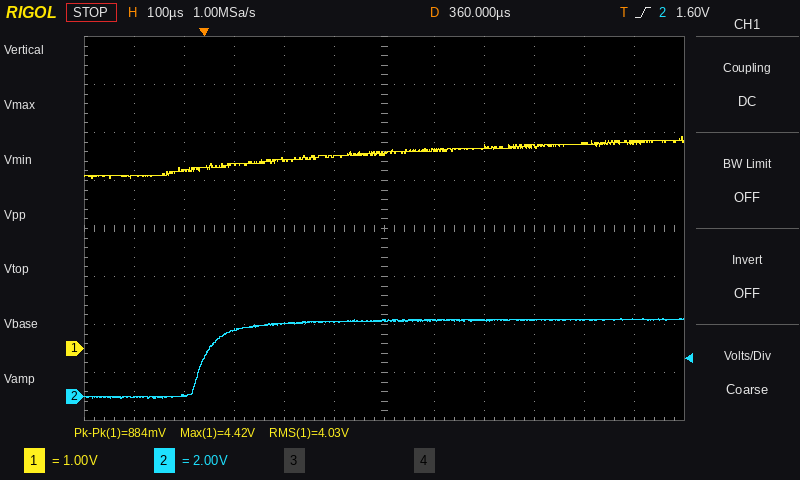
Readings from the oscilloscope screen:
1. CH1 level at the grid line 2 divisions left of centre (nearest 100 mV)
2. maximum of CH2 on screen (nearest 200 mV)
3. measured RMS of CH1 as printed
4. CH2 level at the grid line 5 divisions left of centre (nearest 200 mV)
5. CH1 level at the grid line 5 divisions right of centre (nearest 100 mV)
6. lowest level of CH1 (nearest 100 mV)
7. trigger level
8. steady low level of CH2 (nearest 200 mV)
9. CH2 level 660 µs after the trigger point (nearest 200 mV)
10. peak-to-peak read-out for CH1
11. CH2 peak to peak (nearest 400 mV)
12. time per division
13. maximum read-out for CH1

3.9 V
3.2 V
4.03 V
0.0 V
4.3 V
3.5 V
1.60 V
0.0 V
3.2 V
884 mV
3.2 V
100 µs
4.42 V
